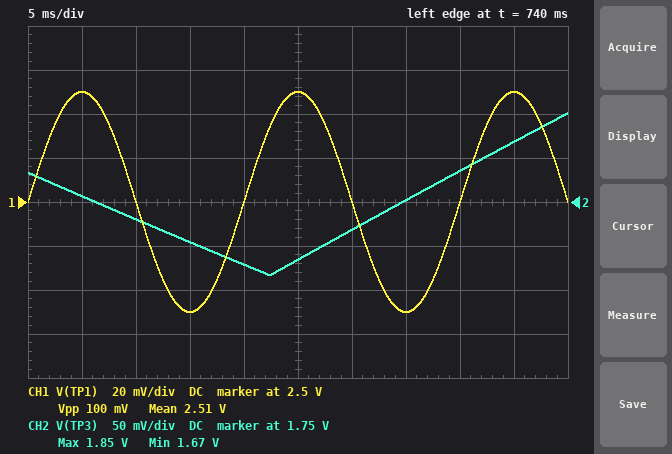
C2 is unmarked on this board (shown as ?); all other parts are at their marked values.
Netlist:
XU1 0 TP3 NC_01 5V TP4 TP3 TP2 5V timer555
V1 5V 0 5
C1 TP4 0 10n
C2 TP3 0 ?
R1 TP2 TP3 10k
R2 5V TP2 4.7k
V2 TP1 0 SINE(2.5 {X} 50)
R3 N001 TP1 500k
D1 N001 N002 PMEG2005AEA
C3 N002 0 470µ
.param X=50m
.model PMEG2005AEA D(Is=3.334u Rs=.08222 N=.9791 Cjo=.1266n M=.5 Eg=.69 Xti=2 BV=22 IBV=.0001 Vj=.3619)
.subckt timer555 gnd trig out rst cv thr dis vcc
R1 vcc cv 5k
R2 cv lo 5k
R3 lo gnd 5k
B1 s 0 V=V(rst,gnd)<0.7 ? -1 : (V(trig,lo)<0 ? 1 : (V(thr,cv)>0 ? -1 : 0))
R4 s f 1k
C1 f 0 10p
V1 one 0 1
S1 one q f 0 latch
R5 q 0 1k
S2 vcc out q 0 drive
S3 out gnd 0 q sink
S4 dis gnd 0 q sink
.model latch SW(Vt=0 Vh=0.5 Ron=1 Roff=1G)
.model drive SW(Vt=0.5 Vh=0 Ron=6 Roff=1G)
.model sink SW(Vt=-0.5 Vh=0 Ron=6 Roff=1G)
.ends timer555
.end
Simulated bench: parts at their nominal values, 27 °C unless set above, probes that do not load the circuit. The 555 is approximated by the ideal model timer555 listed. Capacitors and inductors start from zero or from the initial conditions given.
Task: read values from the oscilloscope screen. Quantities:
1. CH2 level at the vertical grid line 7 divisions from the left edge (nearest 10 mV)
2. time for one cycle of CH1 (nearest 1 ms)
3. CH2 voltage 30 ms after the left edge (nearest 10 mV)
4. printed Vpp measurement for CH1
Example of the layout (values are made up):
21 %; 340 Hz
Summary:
1.75 V; 20 ms; 1.72 V; 100 mV
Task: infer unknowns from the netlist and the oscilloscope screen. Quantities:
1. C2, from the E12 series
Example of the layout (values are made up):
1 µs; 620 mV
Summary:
33 µF
